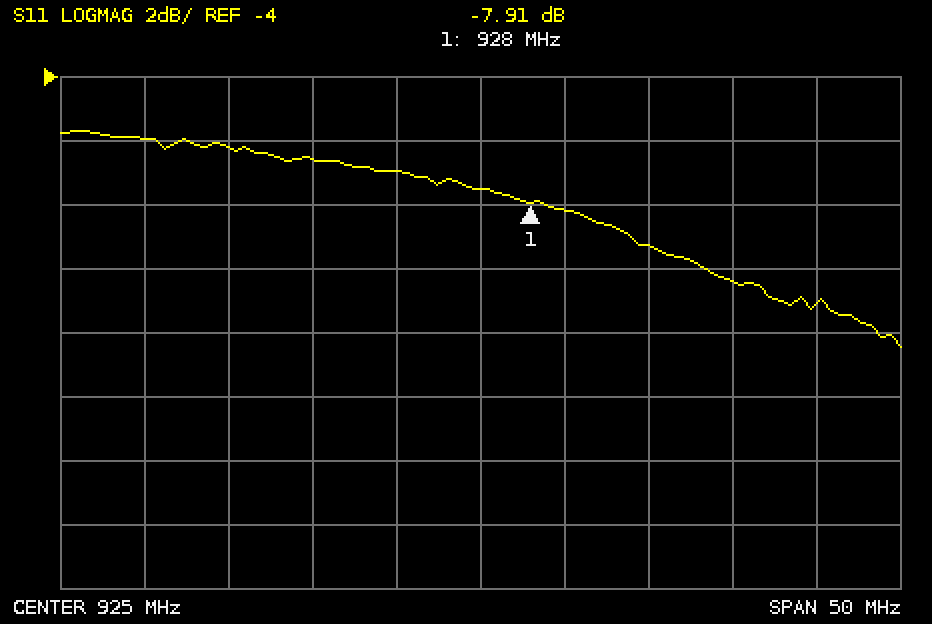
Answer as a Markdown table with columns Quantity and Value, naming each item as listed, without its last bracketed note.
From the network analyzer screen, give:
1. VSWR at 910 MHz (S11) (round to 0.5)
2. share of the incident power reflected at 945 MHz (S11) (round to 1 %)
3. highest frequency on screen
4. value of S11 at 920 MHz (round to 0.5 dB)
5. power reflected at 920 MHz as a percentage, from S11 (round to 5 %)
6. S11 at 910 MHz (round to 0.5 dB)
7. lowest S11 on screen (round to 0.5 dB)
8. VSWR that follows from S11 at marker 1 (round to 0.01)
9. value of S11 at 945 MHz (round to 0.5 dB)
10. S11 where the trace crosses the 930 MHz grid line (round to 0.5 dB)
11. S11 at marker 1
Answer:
| Quantity | Value |
|---|---|
| VSWR at 910 MHz (S11) | 3.0 |
| share of the incident power reflected at 945 MHz (S11) | 8 % |
| highest frequency on screen | 950 MHz |
| value of S11 at 920 MHz | -7.0 dB |
| power reflected at 920 MHz as a percentage, from S11 | 20 % |
| S11 at 910 MHz | -6.0 dB |
| lowest S11 on screen | -12.5 dB |
| VSWR that follows from S11 at marker 1 | 2.35 |
| value of S11 at 945 MHz | -11.0 dB |
| S11 where the trace crosses the 930 MHz grid line | -8.0 dB |
| S11 at marker 1 | -7.91 dB |
